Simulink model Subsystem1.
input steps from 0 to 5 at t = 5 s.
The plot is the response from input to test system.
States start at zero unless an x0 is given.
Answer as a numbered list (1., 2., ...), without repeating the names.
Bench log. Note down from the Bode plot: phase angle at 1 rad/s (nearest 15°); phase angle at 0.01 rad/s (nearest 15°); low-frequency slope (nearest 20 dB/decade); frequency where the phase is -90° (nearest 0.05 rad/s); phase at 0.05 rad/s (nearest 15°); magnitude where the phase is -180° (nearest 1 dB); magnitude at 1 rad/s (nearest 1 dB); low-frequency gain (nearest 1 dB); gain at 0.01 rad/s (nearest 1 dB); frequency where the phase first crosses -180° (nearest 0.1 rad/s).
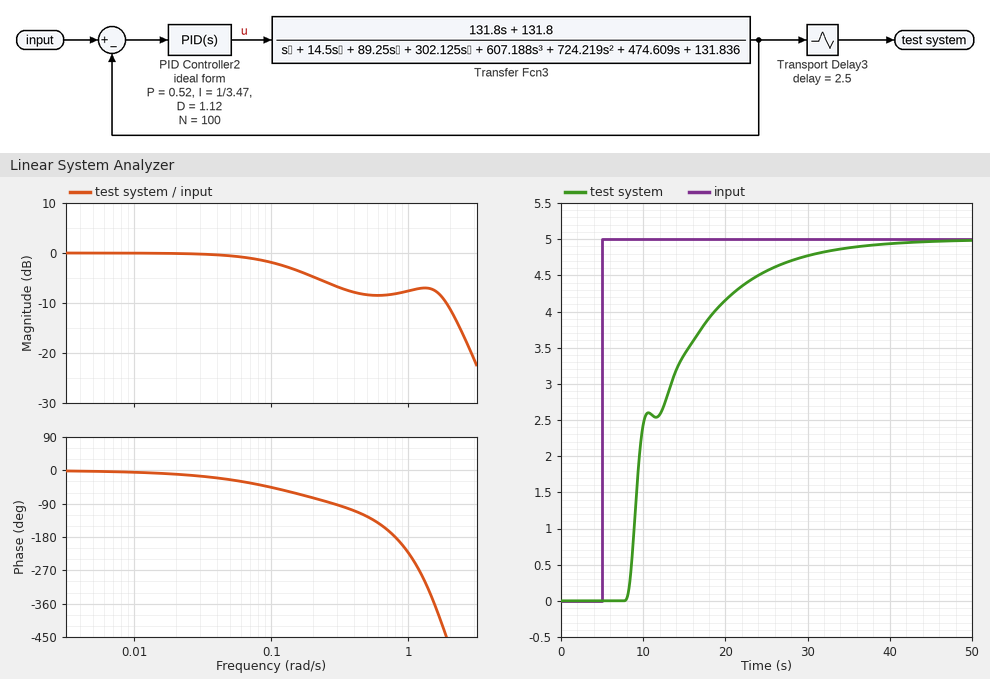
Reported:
1. -225°
2. 0°
3. 0 dB/decade
4. 0.30 rad/s
5. -30°
6. -8 dB
7. -8 dB
8. 0 dB
9. 0 dB
10. 0.8 rad/s
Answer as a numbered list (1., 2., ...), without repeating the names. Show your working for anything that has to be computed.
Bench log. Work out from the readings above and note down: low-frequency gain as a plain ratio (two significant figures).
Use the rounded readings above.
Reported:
1. 10^(0 / 20) = 1.0
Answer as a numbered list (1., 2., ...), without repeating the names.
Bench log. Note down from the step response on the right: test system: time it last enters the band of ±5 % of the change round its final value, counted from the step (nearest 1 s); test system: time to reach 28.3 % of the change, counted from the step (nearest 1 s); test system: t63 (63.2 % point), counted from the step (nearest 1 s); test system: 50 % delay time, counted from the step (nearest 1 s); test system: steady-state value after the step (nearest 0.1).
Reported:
1. 24 s
2. 4 s
3. 9 s
4. 5 s
5. 5.0
